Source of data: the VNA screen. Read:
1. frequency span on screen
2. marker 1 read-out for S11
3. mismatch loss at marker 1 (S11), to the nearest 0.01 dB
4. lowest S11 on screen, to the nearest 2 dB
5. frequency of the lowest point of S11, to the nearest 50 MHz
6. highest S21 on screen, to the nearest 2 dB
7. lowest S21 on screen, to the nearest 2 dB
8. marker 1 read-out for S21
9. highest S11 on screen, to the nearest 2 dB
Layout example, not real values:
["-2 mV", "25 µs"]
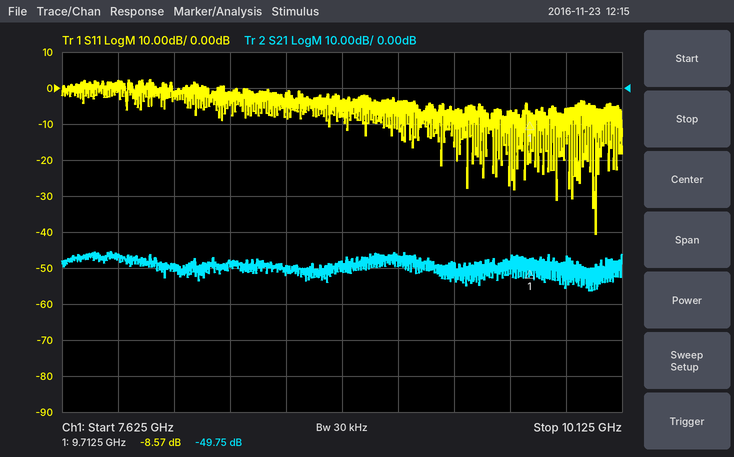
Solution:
["2.5 GHz", "-8.57 dB", "0.65 dB", "-40 dB", "10.00 GHz", "-46 dB", "-56 dB", "-49.75 dB", "2 dB"]
